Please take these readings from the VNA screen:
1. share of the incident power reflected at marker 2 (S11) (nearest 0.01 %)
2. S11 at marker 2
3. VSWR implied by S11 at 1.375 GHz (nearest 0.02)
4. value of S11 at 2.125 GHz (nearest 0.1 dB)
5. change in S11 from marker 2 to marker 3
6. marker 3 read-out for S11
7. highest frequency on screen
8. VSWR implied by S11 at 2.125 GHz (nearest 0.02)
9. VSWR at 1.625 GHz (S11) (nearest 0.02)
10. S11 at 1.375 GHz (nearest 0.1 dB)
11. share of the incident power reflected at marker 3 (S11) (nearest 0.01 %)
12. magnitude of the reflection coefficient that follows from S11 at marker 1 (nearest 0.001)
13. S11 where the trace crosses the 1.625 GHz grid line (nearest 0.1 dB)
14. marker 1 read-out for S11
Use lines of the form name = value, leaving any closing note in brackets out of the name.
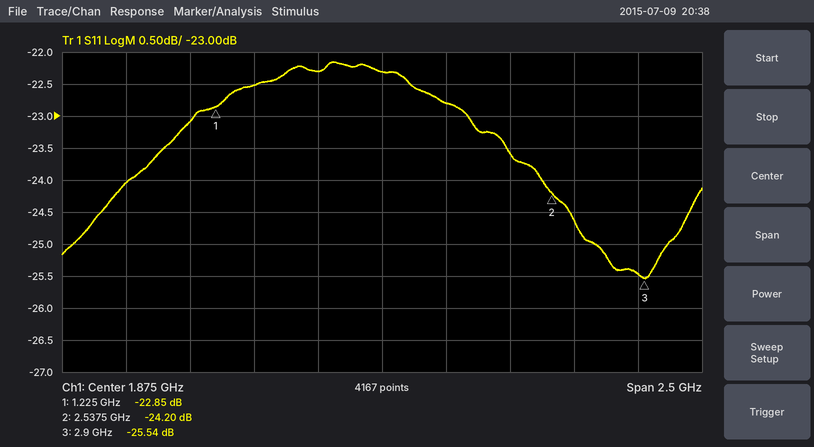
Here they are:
share of the incident power reflected at marker 2 (S11) = 0.38 %
S11 at marker 2 = -24.20 dB
VSWR implied by S11 at 1.375 GHz = 1.16
value of S11 at 2.125 GHz = -22.8 dB
change in S11 from marker 2 to marker 3 = -1.34 dB
marker 3 read-out for S11 = -25.54 dB
highest frequency on screen = 3.125 GHz
VSWR implied by S11 at 2.125 GHz = 1.16
VSWR at 1.625 GHz (S11) = 1.16
S11 at 1.375 GHz = -22.5 dB
share of the incident power reflected at marker 3 (S11) = 0.28 %
magnitude of the reflection coefficient that follows from S11 at marker 1 = 0.072
S11 where the trace crosses the 1.625 GHz grid line = -22.3 dB
marker 1 read-out for S11 = -22.85 dB
